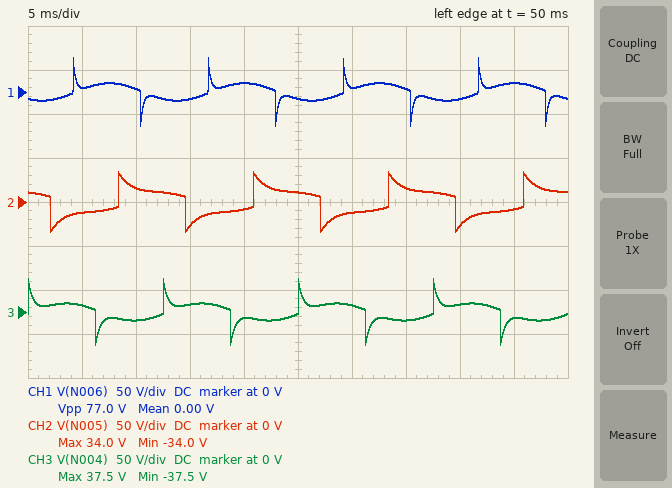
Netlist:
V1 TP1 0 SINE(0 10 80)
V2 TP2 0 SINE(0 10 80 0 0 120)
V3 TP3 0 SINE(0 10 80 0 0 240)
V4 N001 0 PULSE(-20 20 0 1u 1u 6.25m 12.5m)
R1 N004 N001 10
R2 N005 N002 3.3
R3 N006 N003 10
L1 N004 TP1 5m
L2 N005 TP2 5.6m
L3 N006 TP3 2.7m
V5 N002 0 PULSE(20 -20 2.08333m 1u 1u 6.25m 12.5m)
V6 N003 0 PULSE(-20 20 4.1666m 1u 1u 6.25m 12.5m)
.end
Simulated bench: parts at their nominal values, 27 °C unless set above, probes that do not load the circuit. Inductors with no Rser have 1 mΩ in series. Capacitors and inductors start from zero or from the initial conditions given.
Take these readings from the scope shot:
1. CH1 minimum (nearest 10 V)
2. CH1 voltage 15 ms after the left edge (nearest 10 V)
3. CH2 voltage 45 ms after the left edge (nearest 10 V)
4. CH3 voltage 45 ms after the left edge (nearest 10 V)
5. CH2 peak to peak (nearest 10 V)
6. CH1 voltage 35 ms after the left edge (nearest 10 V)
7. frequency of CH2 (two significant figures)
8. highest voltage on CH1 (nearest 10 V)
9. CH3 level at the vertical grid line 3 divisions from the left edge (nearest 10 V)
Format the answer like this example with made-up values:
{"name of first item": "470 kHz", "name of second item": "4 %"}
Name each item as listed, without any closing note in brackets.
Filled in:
{"CH1 minimum": "-40 V", "CH1 voltage 15 ms after the left edge": "-10 V", "CH2 voltage 45 ms after the left edge": "-10 V", "CH3 voltage 45 ms after the left edge": "-10 V", "CH2 peak to peak": "70 V", "CH1 voltage 35 ms after the left edge": "0 V", "frequency of CH2": "80 Hz", "highest voltage on CH1": "40 V", "CH3 level at the vertical grid line 3 divisions from the left edge": "10 V"}
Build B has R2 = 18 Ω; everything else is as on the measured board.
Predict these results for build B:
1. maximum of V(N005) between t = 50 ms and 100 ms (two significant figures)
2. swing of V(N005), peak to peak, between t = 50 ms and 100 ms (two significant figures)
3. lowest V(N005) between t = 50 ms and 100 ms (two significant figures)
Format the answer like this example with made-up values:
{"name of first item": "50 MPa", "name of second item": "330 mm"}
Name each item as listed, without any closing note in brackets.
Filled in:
{"maximum of V(N005) between t = 50 ms and 100 ms": "38 V", "swing of V(N005), peak to peak, between t = 50 ms and 100 ms": "77 V", "lowest V(N005) between t = 50 ms and 100 ms": "-38 V"}
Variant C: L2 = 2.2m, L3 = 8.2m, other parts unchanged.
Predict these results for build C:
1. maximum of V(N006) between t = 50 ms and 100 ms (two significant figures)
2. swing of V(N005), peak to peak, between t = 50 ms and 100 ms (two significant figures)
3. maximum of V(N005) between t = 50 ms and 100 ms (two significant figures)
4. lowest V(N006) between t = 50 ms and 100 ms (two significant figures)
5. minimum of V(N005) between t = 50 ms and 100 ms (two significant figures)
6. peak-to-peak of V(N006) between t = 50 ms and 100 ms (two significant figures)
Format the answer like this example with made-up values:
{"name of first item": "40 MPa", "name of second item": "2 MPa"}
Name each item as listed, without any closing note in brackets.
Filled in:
{"maximum of V(N006) between t = 50 ms and 100 ms": "36 V", "swing of V(N005), peak to peak, between t = 50 ms and 100 ms": "74 V", "maximum of V(N005) between t = 50 ms and 100 ms": "37 V", "lowest V(N006) between t = 50 ms and 100 ms": "-36 V", "minimum of V(N005) between t = 50 ms and 100 ms": "-37 V", "peak-to-peak of V(N006) between t = 50 ms and 100 ms": "73 V"}
